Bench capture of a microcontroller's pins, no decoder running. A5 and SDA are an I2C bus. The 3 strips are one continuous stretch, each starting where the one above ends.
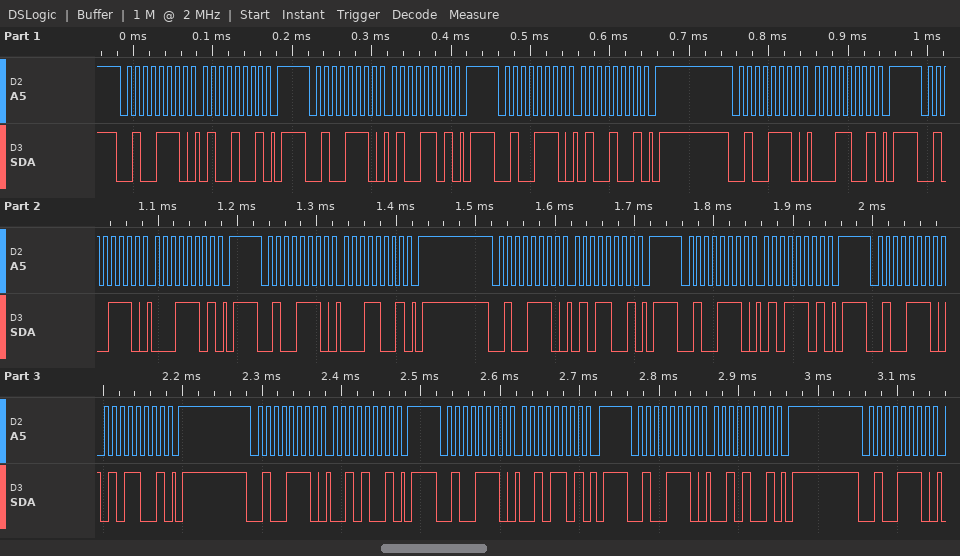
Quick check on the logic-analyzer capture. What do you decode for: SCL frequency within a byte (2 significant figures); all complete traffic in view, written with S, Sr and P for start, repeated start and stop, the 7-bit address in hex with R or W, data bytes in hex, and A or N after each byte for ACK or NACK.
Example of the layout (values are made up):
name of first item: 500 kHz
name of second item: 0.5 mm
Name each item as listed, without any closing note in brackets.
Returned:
SCL frequency within a byte: 100 kHz
all complete traffic in view, written with S, Sr and P for start, repeated start and stop, the 7-bit address in hex with R or W, data bytes in hex, and A or N after each byte for ACK or NACK: S 27W A 49 A P S 27W A 4D A P S 27W A 49 A P S 27W A 19 A P S 27W A 1D A P S 27W A 19 A P S 27W A 59 A P S 27W A 5D A P S 27W A 59 A P S 27W A 29 A P S 27W A 2D A P S 27W A 29 A P S 27W A
